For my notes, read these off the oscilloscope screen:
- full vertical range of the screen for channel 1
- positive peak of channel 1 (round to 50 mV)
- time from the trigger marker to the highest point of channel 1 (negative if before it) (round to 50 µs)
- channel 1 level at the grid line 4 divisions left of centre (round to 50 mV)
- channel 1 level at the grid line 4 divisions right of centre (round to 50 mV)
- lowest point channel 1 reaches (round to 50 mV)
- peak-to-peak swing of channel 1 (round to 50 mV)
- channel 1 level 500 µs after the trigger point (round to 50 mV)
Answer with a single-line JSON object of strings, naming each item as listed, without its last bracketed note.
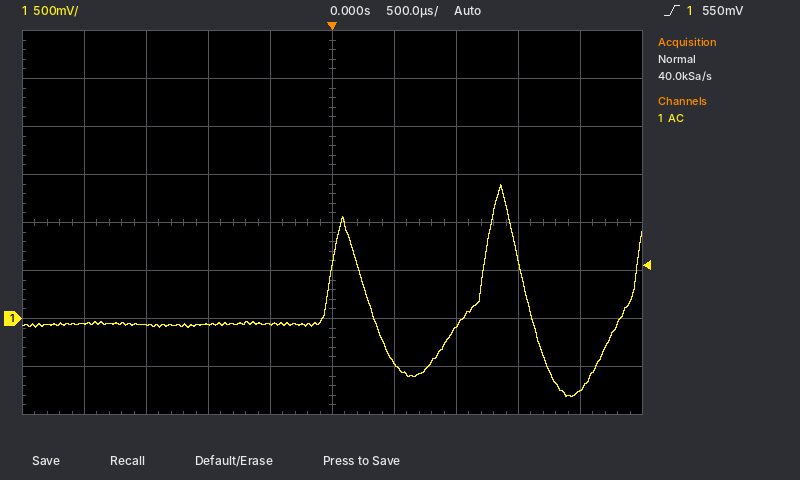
{"full vertical range of the screen for channel 1": "4 V", "positive peak of channel 1": "1.40 V", "time from the trigger marker to the highest point of channel 1 (negative if before it)": "+1.35 ms", "channel 1 level at the grid line 4 divisions left of centre": "-50 mV", "channel 1 level at the grid line 4 divisions right of centre": "-750 mV", "lowest point channel 1 reaches": "-800 mV", "peak-to-peak swing of channel 1": "2.20 V", "channel 1 level 500 µs after the trigger point": "-450 mV"}
